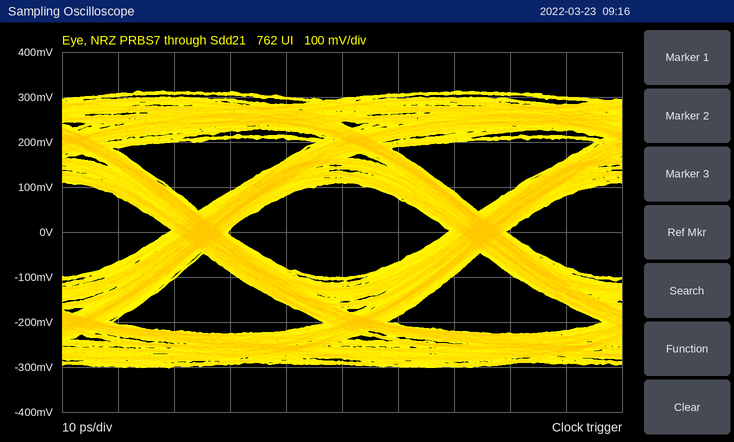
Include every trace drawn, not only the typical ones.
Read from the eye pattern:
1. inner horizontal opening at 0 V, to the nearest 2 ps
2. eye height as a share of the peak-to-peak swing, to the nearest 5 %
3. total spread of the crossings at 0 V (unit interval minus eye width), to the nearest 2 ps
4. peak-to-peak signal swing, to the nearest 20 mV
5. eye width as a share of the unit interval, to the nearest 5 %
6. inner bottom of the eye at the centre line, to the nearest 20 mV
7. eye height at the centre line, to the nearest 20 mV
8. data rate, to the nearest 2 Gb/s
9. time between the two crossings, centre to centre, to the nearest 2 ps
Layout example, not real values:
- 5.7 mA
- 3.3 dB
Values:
- 40 ps
- 35 %
- 10 ps
- 620 mV
- 80 %
- -100 mV
- 220 mV
- 20 Gb/s
- 50 ps
